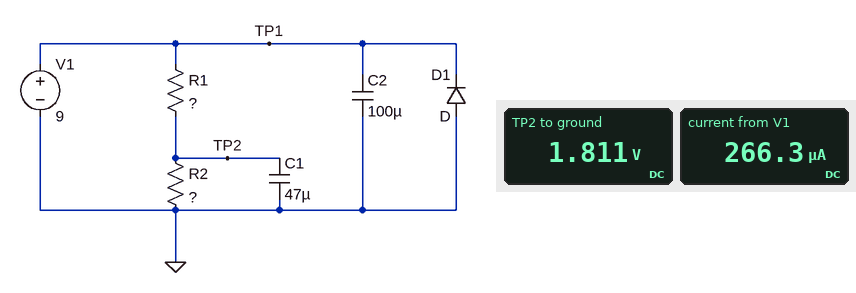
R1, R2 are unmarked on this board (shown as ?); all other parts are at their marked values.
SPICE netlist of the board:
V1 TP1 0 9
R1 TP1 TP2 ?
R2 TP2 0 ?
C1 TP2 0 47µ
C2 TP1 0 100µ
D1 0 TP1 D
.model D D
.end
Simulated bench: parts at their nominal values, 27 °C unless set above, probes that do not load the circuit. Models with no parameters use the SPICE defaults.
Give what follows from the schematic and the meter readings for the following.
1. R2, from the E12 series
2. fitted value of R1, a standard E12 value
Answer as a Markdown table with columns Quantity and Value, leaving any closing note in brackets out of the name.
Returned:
| Quantity | Value |
|---|---|
| R2, from the E12 series | 6.8 kΩ |
| fitted value of R1, a standard E12 value | 27 kΩ |
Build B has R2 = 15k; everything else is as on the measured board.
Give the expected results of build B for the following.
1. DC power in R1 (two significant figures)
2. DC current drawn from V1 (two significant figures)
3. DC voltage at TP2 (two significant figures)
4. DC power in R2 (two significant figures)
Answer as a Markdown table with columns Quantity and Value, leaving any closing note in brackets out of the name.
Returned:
| Quantity | Value |
|---|---|
| DC power in R1 | 1.2 mW |
| DC current drawn from V1 | 210 µA |
| DC voltage at TP2 | 3.2 V |
| DC power in R2 | 690 µW |
